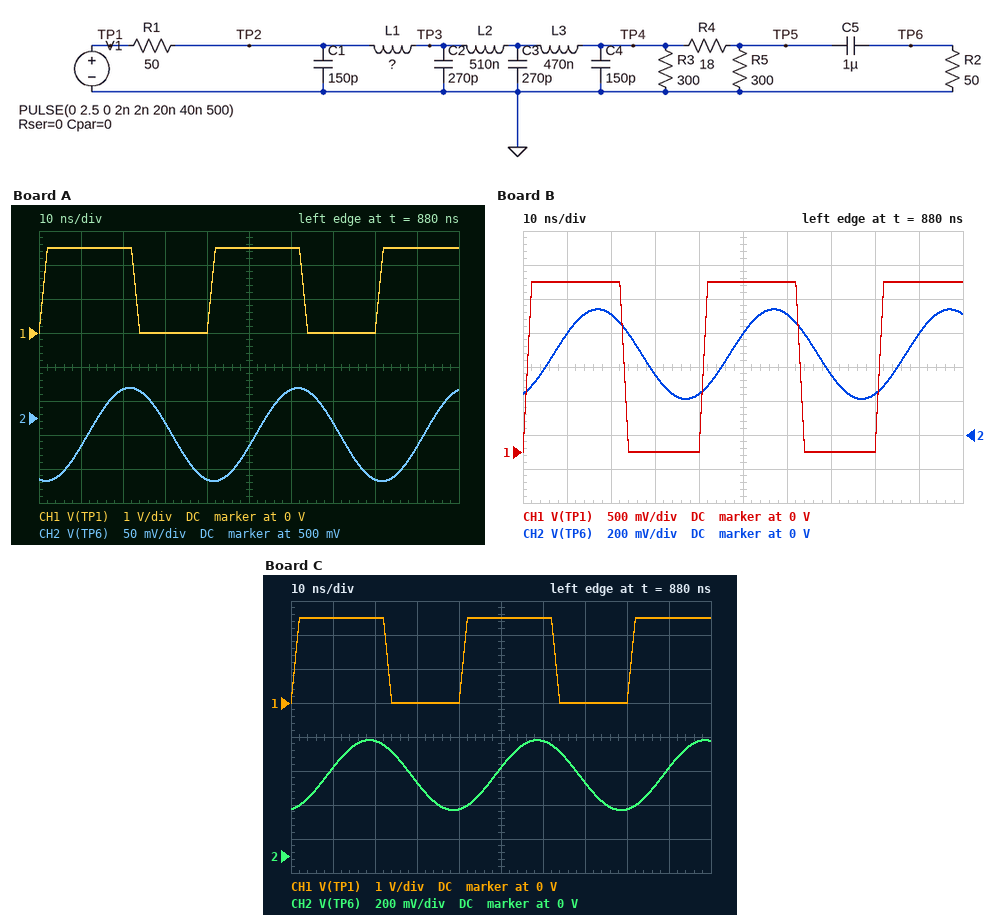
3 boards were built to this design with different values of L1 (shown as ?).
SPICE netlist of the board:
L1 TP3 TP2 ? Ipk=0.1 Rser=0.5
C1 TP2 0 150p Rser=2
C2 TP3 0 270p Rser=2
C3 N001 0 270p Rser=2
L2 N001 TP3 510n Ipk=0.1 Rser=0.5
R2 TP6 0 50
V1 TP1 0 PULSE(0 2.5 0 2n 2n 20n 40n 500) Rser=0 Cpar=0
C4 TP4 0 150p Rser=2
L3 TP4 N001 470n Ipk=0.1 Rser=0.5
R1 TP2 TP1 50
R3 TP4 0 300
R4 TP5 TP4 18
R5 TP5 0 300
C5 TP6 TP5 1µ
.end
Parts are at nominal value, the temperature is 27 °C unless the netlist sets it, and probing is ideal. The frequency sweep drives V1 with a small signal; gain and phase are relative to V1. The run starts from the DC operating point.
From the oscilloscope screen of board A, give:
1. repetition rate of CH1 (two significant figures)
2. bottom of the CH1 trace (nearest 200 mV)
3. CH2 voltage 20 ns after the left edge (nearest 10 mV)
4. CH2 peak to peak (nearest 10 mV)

25 MHz
0 V
540 mV
140 mV
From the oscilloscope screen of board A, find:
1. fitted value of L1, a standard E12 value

1.5 µH
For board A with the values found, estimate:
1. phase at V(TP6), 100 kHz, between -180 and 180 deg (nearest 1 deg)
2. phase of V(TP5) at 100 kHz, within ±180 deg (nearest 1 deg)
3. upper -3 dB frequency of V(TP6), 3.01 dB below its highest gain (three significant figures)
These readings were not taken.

-1 deg
-3 deg
11.0 MHz
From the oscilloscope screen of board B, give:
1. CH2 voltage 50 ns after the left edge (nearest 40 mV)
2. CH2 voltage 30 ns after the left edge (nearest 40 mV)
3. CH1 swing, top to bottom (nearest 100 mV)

600 mV
360 mV
2.5 V
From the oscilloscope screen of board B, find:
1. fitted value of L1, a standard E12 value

560 nH
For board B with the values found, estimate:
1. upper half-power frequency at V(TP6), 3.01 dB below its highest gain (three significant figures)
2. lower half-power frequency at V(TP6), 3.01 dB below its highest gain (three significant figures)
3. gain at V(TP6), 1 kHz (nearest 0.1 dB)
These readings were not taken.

21.9 MHz
1.57 kHz
-14.5 dB
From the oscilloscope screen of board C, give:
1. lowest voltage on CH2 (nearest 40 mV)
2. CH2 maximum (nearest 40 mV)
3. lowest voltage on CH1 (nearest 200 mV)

280 mV
680 mV
0 V
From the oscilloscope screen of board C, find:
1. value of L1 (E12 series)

680 nH
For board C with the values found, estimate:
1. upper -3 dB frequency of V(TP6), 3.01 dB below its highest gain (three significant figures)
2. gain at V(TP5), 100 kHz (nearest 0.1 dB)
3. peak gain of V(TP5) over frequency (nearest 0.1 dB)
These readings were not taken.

20.0 MHz
-9.1 dB
-3.0 dB
